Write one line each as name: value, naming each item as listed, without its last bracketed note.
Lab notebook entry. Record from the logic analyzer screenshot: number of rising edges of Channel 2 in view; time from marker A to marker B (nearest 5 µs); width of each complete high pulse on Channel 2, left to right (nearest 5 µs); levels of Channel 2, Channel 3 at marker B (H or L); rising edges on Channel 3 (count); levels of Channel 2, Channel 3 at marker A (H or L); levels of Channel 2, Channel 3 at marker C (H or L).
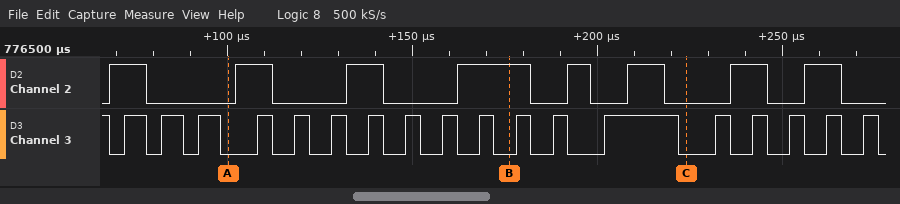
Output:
number of rising edges of Channel 2 in view: 8
time from marker A to marker B: 75 µs
width of each complete high pulse on Channel 2, left to right: 10 µs, 10 µs, 10 µs, 20 µs, 5 µs, 10 µs, 10 µs, 10 µs
levels of Channel 2, Channel 3 at marker B: Channel 2=H, Channel 3=L
rising edges on Channel 3: 18
levels of Channel 2, Channel 3 at marker A: Channel 2=L, Channel 3=L
levels of Channel 2, Channel 3 at marker C: Channel 2=L, Channel 3=L
